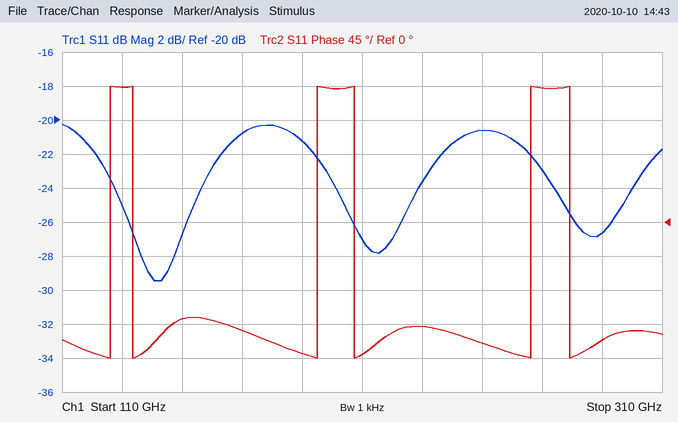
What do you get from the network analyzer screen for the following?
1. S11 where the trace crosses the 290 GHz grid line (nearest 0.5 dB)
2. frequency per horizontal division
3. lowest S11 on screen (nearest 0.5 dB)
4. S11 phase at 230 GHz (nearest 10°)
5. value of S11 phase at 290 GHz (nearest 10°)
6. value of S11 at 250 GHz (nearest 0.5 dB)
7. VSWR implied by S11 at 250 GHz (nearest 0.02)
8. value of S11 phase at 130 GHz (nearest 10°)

-26.5 dB
20 GHz
-29.5 dB
-140°
-160°
-20.5 dB
1.20
180°
